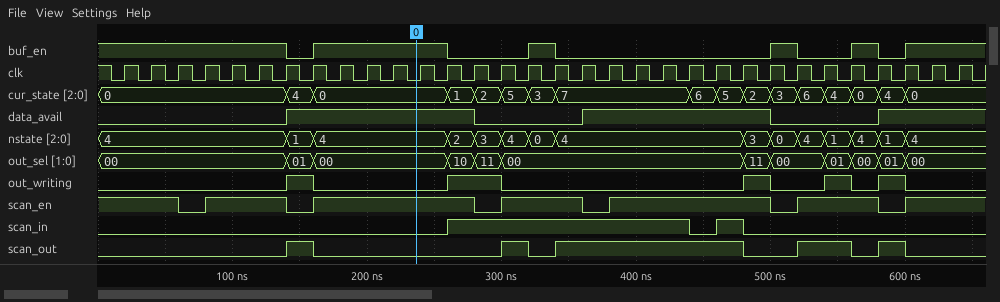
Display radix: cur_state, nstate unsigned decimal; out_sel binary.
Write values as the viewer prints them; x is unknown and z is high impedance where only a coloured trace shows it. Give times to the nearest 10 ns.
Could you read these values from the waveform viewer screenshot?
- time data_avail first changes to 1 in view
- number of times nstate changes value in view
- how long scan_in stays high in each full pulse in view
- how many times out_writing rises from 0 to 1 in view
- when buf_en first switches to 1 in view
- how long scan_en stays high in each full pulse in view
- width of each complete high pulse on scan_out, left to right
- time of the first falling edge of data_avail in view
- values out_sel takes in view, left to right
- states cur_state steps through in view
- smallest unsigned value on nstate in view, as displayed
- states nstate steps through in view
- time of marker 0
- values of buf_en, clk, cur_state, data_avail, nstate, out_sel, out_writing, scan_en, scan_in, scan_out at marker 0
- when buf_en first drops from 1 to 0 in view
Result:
140 ns
14
180 ns, 20 ns
5
160 ns
60 ns, 120 ns, 60 ns, 120 ns, 60 ns
20 ns, 20 ns, 140 ns, 40 ns, 20 ns
280 ns
00, 01, 00, 10, 11, 00, 11, 00, 01, 00, 01, 00
0, 4, 0, 1, 2, 5, 3, 7, 6, 5, 2, 3, 6, 4, 0, 4, 0
0
4, 1, 4, 2, 3, 4, 0, 4, 3, 0, 4, 1, 4, 1, 4
240 ns
buf_en=1, clk=0, cur_state=0, data_avail=1, nstate=4, out_sel=00, out_writing=0, scan_en=1, scan_in=0, scan_out=0
140 ns
